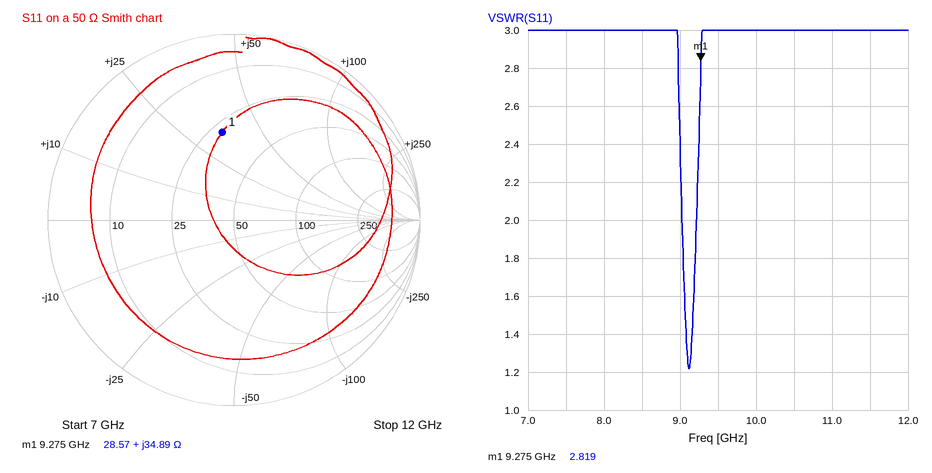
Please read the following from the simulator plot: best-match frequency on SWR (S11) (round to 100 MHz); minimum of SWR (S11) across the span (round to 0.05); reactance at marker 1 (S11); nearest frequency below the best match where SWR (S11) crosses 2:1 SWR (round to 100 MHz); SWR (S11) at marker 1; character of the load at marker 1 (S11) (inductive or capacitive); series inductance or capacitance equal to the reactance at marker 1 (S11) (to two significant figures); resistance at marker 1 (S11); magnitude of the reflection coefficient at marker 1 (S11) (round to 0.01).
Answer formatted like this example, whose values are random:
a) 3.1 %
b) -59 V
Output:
a) 9.1 GHz
b) 1.20
c) +34.89 Ω
d) 9.0 GHz
e) 2.819
f) inductive
g) 600 pH
h) 28.57 Ω
i) 0.48
